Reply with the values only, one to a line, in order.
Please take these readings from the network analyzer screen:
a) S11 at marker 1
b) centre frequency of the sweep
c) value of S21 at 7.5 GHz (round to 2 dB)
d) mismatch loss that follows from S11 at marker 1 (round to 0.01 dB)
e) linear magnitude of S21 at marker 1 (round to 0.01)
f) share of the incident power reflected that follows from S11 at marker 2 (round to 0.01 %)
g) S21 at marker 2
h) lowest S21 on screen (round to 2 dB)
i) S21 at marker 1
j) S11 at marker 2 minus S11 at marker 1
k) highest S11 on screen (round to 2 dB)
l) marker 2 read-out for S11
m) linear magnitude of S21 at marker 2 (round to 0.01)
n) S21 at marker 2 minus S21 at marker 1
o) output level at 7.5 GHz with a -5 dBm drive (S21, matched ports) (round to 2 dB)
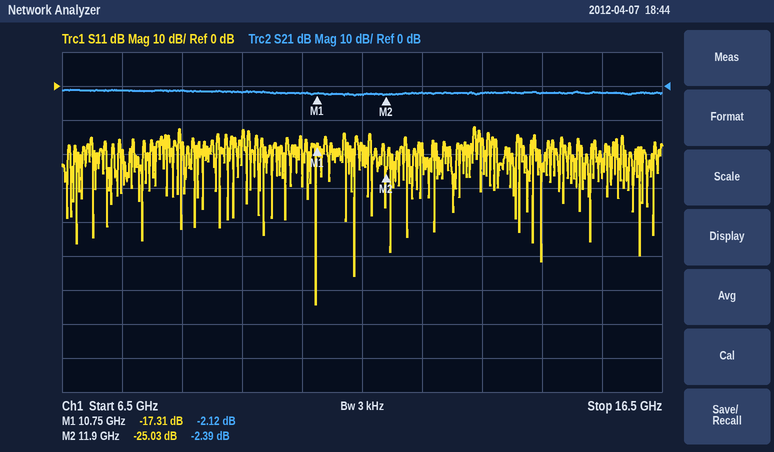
-17.31 dB
11.5 GHz
-2 dB
0.08 dB
0.78
0.31 %
-2.39 dB
-2 dB
-2.12 dB
-7.72 dB
-12 dB
-25.03 dB
0.76
-0.27 dB
-6 dBm
